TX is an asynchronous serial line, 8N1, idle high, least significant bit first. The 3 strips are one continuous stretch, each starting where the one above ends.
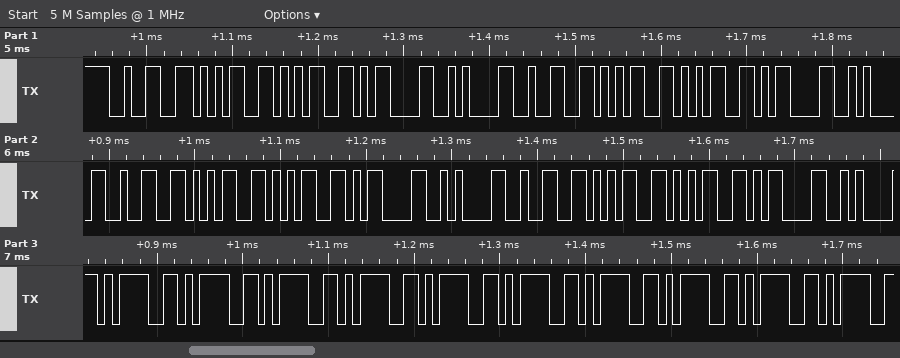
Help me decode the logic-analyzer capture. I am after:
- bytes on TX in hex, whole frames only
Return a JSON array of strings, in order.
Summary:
["0x32 0x35 0x35 0x0D 0x0A 0x32 0x35 0x35 0x0D 0x0A 0x32 0x35 0x35 0x0D 0x0A 0x32 0x35 0x35 0x0D 0x0A 0x3D 0x3D 0x3D 0x3D 0x3D 0x3D 0x3D 0x3D 0x3D 0x3D"]
